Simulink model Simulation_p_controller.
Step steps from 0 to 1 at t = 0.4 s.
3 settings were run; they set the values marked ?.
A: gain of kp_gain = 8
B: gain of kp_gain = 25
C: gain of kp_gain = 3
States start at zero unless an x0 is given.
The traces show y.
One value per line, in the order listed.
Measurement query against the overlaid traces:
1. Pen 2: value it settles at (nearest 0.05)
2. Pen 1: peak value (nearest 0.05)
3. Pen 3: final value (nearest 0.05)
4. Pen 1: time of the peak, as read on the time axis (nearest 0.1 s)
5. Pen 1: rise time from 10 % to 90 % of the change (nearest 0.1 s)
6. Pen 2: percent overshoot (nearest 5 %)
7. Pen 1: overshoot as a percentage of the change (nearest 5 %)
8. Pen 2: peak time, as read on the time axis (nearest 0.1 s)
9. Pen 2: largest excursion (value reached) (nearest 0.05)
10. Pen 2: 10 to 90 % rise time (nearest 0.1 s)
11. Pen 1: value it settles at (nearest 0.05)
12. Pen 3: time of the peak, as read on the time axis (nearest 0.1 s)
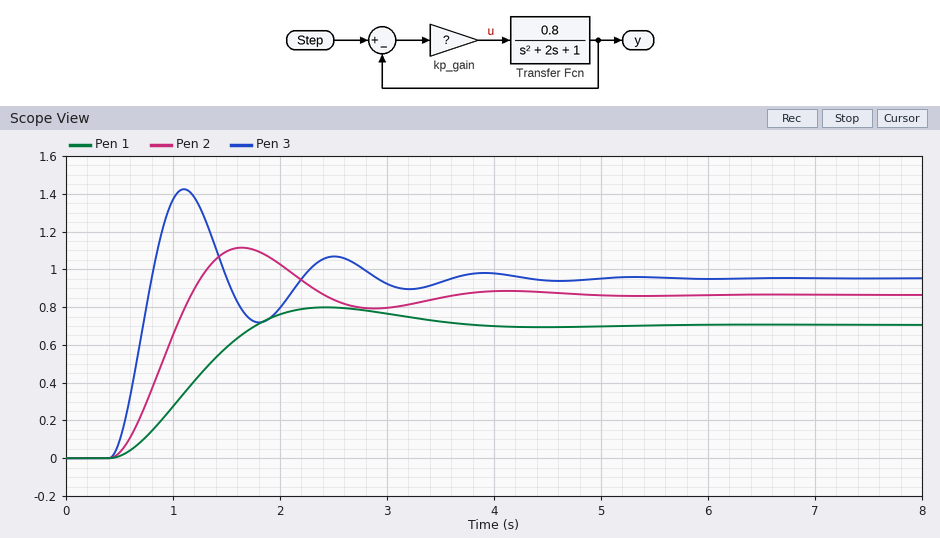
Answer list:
0.85
0.80
0.95
2.4 s
0.9 s
30 %
15 %
1.6 s
1.10
0.5 s
0.70
1.1 s
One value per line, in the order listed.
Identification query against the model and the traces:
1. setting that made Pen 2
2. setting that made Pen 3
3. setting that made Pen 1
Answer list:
A
B
C
